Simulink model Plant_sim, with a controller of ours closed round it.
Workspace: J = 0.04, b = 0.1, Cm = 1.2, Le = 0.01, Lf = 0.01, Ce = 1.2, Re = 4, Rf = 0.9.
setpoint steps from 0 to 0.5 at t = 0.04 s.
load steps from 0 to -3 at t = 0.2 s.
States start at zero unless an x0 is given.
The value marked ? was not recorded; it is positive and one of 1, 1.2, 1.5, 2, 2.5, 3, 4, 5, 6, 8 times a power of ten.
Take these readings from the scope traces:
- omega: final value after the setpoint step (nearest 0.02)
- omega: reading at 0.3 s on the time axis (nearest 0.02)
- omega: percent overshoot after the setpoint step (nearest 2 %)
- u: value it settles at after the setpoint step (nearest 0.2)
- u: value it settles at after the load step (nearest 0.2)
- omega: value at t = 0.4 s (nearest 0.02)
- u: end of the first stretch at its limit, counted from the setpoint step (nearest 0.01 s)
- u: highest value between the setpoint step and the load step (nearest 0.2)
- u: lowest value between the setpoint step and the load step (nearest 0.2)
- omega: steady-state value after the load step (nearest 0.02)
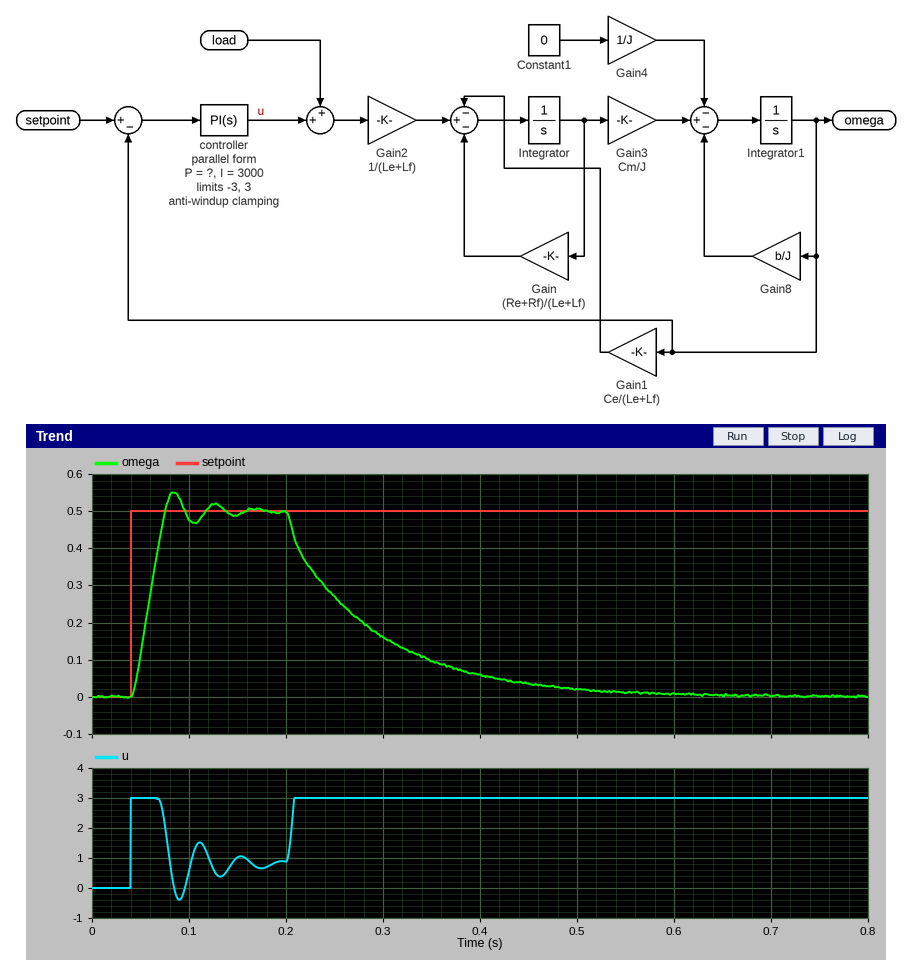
0.50
0.16
10 %
0.8
3.0
0.06
0.03 s
3.0
-0.4
0.00
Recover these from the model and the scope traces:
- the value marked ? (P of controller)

20
